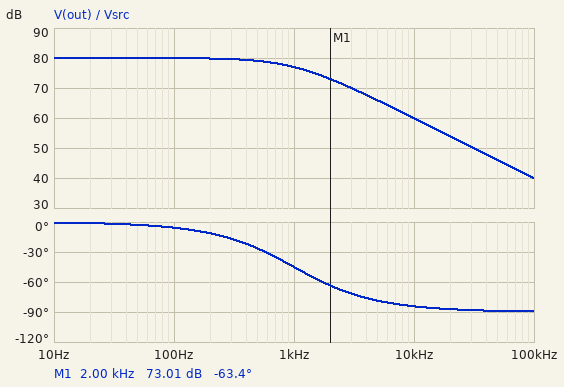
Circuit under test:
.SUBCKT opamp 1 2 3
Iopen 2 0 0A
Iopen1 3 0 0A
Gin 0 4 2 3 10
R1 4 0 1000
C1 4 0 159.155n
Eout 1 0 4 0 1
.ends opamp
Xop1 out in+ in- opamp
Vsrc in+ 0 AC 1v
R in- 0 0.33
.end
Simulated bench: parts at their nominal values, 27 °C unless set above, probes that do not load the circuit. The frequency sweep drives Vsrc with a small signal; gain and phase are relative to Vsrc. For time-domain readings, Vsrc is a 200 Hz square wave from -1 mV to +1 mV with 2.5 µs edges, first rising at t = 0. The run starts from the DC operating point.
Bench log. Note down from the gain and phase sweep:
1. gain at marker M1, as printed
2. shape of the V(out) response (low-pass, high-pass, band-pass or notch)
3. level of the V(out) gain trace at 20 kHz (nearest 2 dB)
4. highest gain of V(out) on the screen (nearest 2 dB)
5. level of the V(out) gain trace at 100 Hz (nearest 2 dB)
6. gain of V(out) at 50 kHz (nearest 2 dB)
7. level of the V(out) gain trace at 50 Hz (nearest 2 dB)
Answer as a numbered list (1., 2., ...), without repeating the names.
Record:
1. 73.01 dB
2. low-pass
3. 54 dB
4. 80 dB
5. 80 dB
6. 46 dB
7. 80 dB
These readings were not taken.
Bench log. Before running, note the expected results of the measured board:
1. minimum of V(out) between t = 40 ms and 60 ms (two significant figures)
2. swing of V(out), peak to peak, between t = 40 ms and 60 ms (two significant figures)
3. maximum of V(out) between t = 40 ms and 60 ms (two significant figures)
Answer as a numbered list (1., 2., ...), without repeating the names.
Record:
1. -10 V
2. 20 V
3. 10 V
